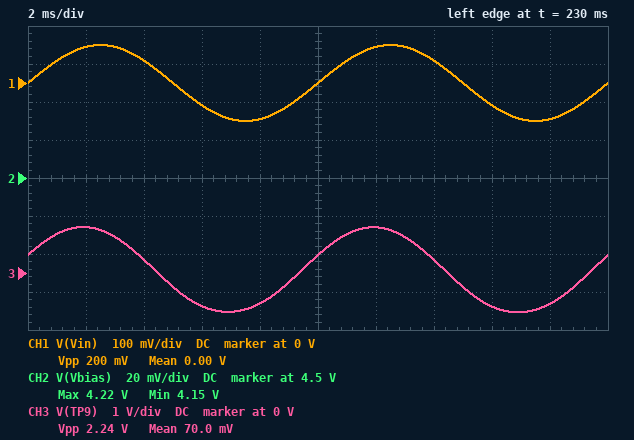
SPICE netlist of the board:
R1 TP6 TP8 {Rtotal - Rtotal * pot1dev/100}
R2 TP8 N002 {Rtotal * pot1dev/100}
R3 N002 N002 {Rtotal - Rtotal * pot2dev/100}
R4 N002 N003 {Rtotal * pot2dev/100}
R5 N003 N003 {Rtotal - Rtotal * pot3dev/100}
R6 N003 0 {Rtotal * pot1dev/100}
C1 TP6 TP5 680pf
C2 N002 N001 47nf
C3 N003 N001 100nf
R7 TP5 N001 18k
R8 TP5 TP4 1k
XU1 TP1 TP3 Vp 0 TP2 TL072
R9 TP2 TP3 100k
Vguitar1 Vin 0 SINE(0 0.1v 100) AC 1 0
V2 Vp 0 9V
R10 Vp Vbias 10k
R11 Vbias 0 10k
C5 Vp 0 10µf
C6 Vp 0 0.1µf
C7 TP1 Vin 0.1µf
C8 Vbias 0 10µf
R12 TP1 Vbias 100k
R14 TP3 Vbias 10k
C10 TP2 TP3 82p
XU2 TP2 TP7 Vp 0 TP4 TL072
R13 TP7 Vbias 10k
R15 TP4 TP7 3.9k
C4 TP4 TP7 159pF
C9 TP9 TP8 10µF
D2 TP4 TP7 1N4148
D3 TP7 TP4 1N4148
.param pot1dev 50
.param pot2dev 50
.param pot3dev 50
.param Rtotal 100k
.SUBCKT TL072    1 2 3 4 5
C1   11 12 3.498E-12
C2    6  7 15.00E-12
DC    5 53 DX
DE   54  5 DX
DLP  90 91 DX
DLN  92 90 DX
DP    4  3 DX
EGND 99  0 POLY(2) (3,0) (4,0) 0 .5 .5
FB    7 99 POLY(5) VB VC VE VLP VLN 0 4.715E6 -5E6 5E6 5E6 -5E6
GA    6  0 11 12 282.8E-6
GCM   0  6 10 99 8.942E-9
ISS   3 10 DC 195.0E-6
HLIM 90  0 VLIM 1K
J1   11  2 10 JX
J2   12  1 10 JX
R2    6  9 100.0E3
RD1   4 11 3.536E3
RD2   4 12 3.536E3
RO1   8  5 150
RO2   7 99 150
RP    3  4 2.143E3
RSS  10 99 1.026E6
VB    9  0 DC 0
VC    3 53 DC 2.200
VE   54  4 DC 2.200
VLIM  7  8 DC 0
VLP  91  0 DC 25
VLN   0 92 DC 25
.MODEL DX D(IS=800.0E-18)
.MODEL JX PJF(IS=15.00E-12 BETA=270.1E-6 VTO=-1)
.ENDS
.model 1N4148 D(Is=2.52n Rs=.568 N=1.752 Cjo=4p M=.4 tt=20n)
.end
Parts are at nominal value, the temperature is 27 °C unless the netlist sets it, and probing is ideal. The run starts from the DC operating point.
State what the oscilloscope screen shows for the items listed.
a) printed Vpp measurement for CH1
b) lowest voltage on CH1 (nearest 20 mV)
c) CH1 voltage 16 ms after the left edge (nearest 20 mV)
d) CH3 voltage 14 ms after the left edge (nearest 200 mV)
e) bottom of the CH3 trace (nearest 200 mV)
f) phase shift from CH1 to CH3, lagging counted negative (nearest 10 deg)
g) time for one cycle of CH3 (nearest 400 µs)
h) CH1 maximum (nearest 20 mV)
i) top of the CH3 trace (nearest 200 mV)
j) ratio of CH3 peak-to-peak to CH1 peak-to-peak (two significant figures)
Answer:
200 mV
-100 mV
-60 mV
400 mV
-1.0 V
20 deg
10.0 ms
100 mV
1.2 V
11
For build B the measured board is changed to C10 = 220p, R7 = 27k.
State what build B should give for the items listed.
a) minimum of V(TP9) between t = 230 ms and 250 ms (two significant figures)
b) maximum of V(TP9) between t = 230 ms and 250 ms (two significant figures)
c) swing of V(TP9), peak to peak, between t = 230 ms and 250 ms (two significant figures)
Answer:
-920 mV
1.1 V
2.0 V
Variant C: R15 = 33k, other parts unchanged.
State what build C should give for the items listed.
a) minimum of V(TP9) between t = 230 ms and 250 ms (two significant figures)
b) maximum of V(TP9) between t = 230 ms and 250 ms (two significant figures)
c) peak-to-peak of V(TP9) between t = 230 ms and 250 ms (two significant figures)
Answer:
-1.1 V
1.4 V
2.5 V
